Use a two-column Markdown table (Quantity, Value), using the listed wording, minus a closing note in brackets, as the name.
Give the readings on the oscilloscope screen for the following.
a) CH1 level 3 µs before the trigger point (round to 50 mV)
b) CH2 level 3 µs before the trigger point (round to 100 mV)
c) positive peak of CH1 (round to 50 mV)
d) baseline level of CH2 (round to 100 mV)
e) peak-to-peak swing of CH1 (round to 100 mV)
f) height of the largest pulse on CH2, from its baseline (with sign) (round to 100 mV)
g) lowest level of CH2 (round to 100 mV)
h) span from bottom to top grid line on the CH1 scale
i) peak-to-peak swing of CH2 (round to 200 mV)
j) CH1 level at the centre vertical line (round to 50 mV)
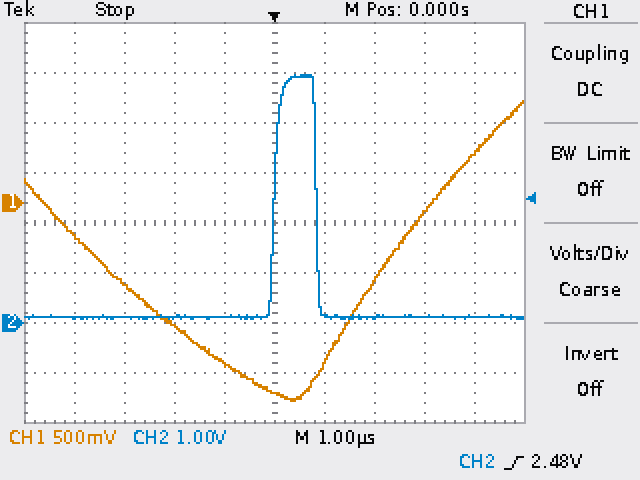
| Quantity | Value |
|---|---|
| CH1 level 3 µs before the trigger point | -800 mV |
| CH2 level 3 µs before the trigger point | 100 mV |
| positive peak of CH1 | 1.00 V |
| baseline level of CH2 | 100 mV |
| peak-to-peak swing of CH1 | 3.00 V |
| height of the largest pulse on CH2, from its baseline (with sign) | +4.8 V |
| lowest level of CH2 | 100 mV |
| span from bottom to top grid line on the CH1 scale | 4 V |
| peak-to-peak swing of CH2 | 4.8 V |
| CH1 level at the centre vertical line | -1.90 V |
